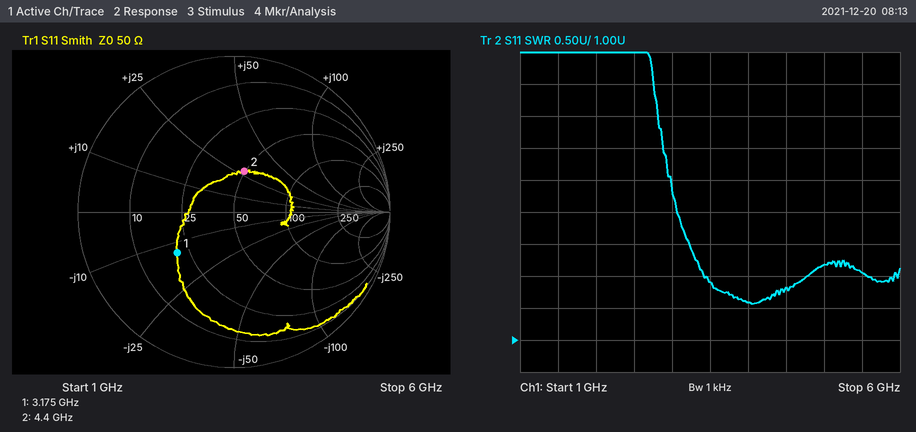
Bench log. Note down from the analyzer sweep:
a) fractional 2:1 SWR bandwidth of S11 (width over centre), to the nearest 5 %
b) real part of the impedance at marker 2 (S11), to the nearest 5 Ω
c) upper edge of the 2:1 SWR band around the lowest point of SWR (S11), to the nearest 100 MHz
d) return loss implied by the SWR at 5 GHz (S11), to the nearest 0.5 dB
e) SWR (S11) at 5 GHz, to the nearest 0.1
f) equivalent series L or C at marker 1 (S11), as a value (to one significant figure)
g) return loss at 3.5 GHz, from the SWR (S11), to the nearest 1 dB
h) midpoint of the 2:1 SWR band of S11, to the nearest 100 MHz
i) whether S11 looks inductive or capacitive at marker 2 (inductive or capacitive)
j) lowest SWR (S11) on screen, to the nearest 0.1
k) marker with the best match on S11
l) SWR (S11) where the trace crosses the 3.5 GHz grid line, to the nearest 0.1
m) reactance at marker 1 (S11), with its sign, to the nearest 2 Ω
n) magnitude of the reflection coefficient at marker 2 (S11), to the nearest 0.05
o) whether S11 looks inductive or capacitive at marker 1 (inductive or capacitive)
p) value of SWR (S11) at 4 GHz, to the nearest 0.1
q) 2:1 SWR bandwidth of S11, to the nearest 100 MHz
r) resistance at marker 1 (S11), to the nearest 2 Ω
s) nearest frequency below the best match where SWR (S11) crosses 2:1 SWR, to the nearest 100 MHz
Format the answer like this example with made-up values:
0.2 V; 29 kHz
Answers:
35 %; 50 Ω; 4.8 GHz; 8.5 dB; 2.2; 4 pF; 10 dB; 4.1 GHz; inductive; 1.6; marker 2; 1.9; -14 Ω; 0.25; capacitive; 1.6; 1.4 GHz; 20 Ω; 3.4 GHz
